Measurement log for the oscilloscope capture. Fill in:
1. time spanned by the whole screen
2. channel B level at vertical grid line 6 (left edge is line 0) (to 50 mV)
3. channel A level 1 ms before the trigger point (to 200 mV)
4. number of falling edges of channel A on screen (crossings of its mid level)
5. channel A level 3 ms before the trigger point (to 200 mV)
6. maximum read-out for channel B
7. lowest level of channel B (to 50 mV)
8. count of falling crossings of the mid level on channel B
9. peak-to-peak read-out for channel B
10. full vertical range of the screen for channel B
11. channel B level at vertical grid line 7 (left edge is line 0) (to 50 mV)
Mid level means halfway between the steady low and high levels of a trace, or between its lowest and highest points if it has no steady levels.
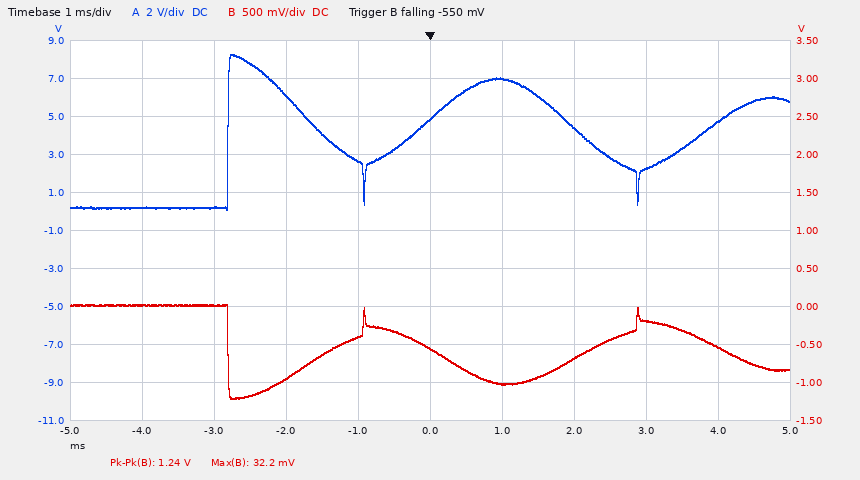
10 ms
-1.00 V
2.6 V
2
200 mV
32.2 mV
-1.20 V
3
1.24 V
5 V
-700 mV
